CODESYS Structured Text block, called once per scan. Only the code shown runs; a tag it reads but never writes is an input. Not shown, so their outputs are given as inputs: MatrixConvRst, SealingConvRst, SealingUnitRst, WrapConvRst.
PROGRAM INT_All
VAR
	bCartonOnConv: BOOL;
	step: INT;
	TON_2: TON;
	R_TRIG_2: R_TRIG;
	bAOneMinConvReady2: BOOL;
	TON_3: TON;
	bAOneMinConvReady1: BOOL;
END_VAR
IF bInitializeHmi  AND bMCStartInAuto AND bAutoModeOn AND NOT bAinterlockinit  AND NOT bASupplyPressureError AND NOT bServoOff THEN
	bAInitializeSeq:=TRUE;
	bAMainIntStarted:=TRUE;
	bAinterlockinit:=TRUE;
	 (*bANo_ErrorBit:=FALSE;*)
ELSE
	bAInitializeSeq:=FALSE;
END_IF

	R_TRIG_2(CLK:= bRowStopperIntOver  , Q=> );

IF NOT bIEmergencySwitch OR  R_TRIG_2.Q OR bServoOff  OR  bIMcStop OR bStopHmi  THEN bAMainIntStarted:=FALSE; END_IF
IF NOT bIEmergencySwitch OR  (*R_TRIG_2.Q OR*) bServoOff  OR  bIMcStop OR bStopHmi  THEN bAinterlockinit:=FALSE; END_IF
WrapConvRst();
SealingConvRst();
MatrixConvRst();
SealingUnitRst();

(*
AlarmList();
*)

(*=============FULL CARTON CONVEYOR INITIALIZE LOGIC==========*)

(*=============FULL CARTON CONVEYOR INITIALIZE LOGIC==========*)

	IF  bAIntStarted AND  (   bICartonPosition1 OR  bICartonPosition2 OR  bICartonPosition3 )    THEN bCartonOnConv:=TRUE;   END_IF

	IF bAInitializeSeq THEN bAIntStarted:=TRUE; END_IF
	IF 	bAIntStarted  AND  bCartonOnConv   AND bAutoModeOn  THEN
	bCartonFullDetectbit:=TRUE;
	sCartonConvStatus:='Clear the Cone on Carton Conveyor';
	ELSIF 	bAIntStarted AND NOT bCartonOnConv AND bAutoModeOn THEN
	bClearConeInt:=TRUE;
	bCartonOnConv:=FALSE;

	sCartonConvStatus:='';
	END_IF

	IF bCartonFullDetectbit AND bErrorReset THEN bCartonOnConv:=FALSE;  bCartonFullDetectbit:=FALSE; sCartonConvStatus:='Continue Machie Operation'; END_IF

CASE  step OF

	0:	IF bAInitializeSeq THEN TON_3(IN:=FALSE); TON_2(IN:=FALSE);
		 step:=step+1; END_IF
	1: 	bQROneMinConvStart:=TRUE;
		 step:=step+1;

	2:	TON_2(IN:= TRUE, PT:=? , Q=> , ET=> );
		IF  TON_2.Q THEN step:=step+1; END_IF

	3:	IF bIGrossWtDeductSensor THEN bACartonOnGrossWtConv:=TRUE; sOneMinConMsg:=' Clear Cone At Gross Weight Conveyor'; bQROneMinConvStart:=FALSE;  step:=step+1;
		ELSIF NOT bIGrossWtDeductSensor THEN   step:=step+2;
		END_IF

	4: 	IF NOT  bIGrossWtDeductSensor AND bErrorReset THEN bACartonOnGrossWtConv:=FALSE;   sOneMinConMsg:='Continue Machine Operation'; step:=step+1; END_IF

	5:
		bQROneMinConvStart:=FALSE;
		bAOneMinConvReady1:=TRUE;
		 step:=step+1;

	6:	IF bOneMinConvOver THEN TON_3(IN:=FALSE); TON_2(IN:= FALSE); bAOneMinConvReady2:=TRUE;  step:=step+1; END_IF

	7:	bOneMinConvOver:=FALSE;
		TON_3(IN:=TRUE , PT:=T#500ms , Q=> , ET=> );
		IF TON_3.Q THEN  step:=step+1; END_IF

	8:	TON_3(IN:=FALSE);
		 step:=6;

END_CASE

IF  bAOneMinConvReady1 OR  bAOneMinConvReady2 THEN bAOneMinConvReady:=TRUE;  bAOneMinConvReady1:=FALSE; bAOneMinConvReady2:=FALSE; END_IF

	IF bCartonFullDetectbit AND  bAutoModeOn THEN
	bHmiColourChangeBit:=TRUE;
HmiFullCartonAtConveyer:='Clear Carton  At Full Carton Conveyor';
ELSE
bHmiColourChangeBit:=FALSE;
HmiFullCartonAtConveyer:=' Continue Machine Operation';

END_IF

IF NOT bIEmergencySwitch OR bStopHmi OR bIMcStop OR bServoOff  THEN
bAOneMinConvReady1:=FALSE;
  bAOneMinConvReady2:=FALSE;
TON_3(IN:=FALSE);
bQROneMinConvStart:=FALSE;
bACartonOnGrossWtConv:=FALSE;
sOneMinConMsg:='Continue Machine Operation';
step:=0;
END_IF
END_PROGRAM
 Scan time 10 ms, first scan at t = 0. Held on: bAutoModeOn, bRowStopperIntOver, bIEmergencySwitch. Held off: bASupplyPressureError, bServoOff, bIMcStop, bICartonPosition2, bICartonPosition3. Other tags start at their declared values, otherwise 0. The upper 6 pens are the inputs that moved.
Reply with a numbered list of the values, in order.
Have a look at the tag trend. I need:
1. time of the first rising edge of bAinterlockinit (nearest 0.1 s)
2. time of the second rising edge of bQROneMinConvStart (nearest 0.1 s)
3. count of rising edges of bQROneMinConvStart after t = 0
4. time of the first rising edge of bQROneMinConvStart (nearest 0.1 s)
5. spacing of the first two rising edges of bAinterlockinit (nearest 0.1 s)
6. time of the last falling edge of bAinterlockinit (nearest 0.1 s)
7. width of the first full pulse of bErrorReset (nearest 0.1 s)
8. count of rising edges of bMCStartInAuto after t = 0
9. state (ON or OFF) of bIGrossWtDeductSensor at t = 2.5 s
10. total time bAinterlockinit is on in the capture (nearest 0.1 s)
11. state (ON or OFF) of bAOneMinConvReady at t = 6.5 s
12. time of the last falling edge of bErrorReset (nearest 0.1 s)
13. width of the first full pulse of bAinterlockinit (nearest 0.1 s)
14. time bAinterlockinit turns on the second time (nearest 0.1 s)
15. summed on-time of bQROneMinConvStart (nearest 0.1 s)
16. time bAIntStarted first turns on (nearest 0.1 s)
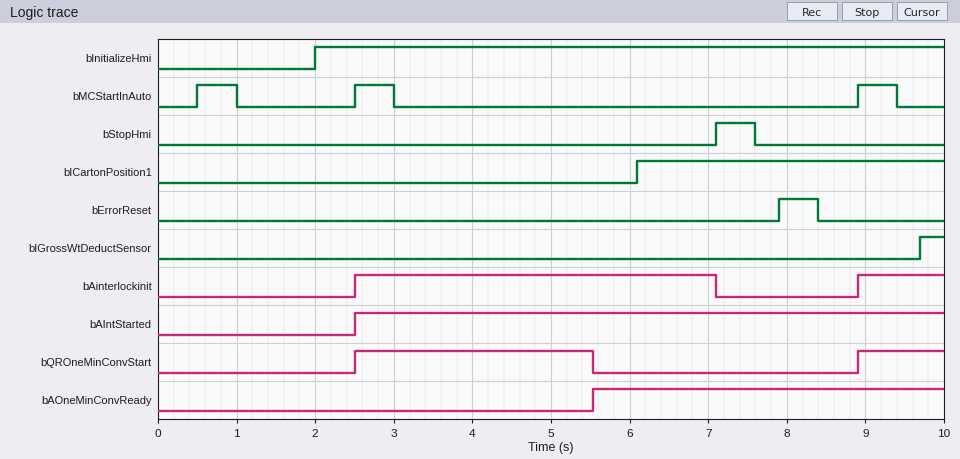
1. 2.5 s
2. 8.9 s
3. 2
4. 2.5 s
5. 6.4 s
6. 7.1 s
7. 0.5 s
8. 3
9. OFF
10. 5.7 s
11. ON
12. 8.4 s
13. 4.6 s
14. 8.9 s
15. 4.1 s
16. 2.5 s
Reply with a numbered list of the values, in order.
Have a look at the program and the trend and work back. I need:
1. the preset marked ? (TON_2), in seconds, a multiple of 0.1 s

1. 3.0 s
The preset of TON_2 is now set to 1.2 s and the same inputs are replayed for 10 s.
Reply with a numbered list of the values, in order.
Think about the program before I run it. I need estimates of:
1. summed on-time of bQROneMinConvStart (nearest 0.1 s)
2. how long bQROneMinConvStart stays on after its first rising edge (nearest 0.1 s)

1. 2.3 s
2. 1.2 s
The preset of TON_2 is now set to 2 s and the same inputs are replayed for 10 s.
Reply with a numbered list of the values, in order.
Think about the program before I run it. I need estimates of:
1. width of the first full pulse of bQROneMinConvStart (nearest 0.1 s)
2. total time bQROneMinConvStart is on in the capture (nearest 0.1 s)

1. 2.0 s
2. 3.1 s
